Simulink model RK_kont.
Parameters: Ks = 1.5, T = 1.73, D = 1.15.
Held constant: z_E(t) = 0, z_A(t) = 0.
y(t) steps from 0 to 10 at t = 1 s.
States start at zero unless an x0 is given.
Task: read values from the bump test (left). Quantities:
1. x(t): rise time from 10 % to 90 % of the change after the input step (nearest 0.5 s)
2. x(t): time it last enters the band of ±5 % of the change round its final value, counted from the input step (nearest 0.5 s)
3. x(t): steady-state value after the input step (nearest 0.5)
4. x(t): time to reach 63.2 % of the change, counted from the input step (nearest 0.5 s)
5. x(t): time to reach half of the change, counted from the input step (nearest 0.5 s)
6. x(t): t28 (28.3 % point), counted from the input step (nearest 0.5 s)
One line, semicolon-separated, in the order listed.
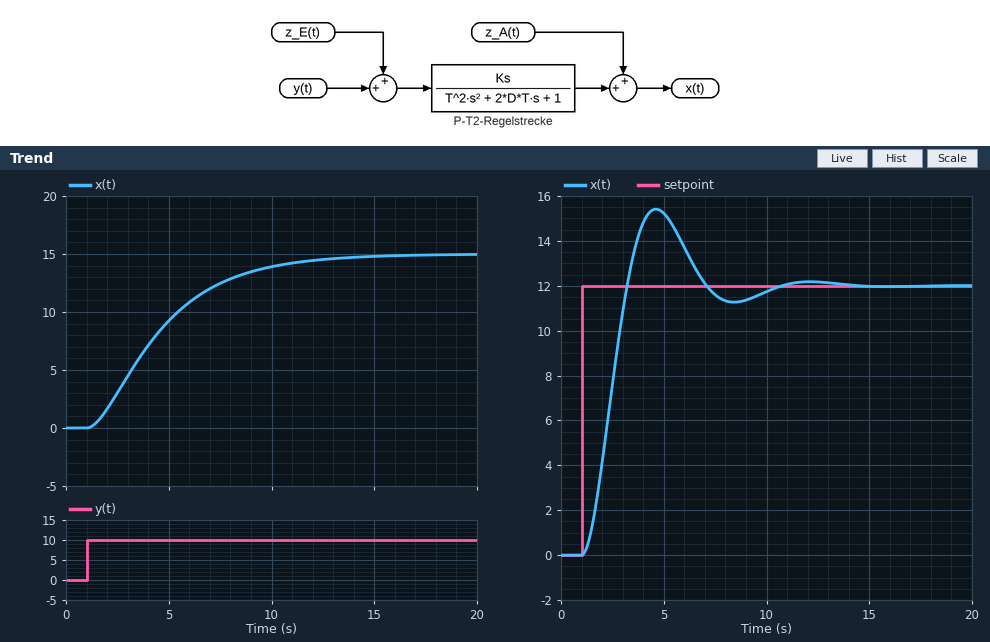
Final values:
7.0 s; 10.0 s; 15.0; 4.0 s; 3.0 s; 2.0 s
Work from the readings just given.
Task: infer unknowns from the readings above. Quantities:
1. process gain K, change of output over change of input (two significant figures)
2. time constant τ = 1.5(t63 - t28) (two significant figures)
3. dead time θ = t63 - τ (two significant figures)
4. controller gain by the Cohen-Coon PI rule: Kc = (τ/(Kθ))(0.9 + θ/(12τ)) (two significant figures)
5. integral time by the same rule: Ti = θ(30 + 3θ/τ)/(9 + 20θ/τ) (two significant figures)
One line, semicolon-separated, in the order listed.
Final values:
1.5; 3.0 s; 1.0 s; 1.9; 2.0 s
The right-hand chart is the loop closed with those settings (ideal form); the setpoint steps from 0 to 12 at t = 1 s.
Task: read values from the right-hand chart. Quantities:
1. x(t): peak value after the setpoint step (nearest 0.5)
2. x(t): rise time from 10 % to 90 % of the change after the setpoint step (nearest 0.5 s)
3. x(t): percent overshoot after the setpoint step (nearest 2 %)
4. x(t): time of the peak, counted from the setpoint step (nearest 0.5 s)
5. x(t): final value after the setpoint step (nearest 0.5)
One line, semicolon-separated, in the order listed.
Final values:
15.5; 1.5 s; 28 %; 3.5 s; 12.0
